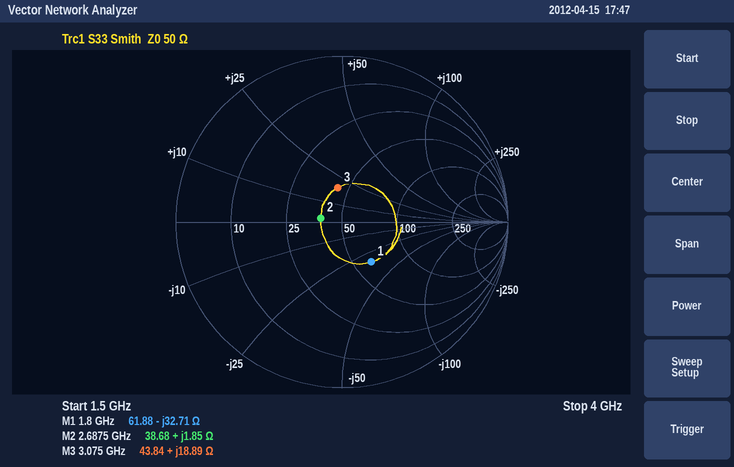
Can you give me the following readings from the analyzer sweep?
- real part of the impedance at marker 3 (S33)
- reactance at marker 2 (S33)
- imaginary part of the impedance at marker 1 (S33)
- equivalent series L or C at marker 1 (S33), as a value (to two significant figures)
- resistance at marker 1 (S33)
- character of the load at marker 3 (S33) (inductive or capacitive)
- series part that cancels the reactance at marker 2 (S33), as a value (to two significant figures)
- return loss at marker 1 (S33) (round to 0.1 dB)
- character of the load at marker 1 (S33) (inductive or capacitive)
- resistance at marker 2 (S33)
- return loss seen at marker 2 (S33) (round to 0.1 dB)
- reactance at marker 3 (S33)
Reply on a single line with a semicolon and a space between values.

43.84 Ω; +1.85 Ω; -32.71 Ω; 2.7 pF; 61.88 Ω; inductive; 32 pF; 10.5 dB; capacitive; 38.68 Ω; 17.8 dB; +18.89 Ω
